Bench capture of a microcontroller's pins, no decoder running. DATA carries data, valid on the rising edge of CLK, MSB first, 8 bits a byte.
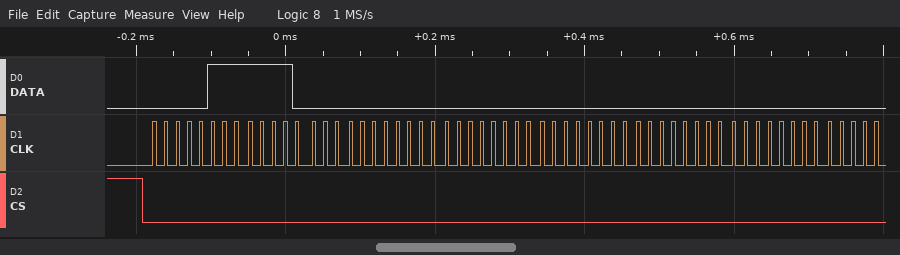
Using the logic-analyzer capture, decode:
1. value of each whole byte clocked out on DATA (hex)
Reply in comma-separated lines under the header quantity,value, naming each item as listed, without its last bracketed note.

quantity,value
value of each whole byte clocked out on DATA,07 F0 00 00 00 00 00
